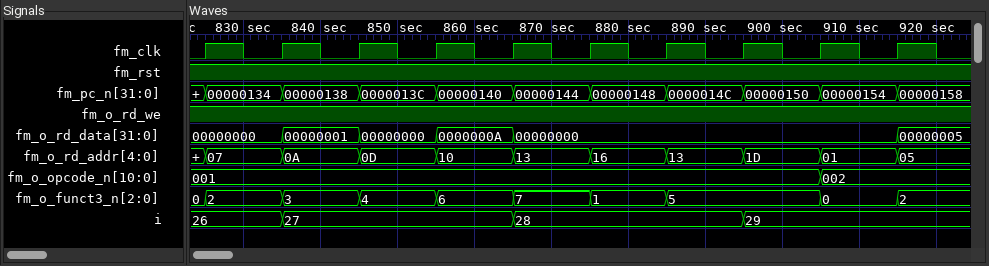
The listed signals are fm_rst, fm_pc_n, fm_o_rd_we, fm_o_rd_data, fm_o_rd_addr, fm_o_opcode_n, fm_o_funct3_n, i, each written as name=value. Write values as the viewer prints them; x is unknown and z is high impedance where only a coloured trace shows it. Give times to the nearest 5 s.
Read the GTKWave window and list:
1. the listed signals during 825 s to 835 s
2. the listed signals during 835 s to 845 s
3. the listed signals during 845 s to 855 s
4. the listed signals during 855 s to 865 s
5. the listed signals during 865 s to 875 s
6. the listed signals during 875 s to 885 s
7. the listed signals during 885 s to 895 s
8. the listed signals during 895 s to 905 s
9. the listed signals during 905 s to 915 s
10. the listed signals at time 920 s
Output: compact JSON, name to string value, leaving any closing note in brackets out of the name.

{"the listed signals during 825 s to 835 s": "fm_rst=1, fm_pc_n=00000134, fm_o_rd_we=1, fm_o_rd_data=00000000, fm_o_rd_addr=07, fm_o_opcode_n=001, fm_o_funct3_n=2, i=26", "the listed signals during 835 s to 845 s": "fm_rst=1, fm_pc_n=00000138, fm_o_rd_we=1, fm_o_rd_data=00000001, fm_o_rd_addr=0A, fm_o_opcode_n=001, fm_o_funct3_n=3, i=27", "the listed signals during 845 s to 855 s": "fm_rst=1, fm_pc_n=0000013C, fm_o_rd_we=1, fm_o_rd_data=00000000, fm_o_rd_addr=0D, fm_o_opcode_n=001, fm_o_funct3_n=4, i=27", "the listed signals during 855 s to 865 s": "fm_rst=1, fm_pc_n=00000140, fm_o_rd_we=1, fm_o_rd_data=0000000A, fm_o_rd_addr=10, fm_o_opcode_n=001, fm_o_funct3_n=6, i=27", "the listed signals during 865 s to 875 s": "fm_rst=1, fm_pc_n=00000144, fm_o_rd_we=1, fm_o_rd_data=00000000, fm_o_rd_addr=13, fm_o_opcode_n=001, fm_o_funct3_n=7, i=28", "the listed signals during 875 s to 885 s": "fm_rst=1, fm_pc_n=00000148, fm_o_rd_we=1, fm_o_rd_data=00000000, fm_o_rd_addr=16, fm_o_opcode_n=001, fm_o_funct3_n=1, i=28", "the listed signals during 885 s to 895 s": "fm_rst=1, fm_pc_n=0000014C, fm_o_rd_we=1, fm_o_rd_data=00000000, fm_o_rd_addr=13, fm_o_opcode_n=001, fm_o_funct3_n=5, i=28", "the listed signals during 895 s to 905 s": "fm_rst=1, fm_pc_n=00000150, fm_o_rd_we=1, fm_o_rd_data=00000000, fm_o_rd_addr=1D, fm_o_opcode_n=001, fm_o_funct3_n=5, i=29", "the listed signals during 905 s to 915 s": "fm_rst=1, fm_pc_n=00000154, fm_o_rd_we=1, fm_o_rd_data=00000000, fm_o_rd_addr=01, fm_o_opcode_n=002, fm_o_funct3_n=0, i=29", "the listed signals at time 920 s": "fm_rst=1, fm_pc_n=00000158, fm_o_rd_we=1, fm_o_rd_data=00000005, fm_o_rd_addr=05, fm_o_opcode_n=002, fm_o_funct3_n=2, i=29"}
